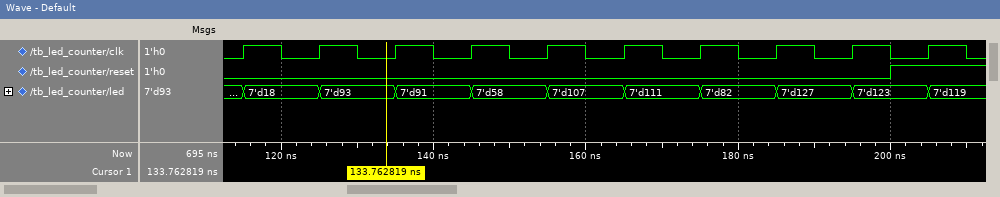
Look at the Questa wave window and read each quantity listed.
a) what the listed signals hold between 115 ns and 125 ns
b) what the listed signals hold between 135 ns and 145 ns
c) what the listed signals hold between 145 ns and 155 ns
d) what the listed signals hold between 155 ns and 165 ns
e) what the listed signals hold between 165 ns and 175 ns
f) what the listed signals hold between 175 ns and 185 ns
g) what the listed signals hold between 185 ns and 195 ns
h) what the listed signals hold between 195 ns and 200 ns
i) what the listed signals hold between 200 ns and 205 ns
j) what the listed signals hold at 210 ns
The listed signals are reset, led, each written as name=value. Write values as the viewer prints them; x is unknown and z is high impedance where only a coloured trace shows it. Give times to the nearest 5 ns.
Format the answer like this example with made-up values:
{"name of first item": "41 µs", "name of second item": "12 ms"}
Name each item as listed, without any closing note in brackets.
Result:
{"what the listed signals hold between 115 ns and 125 ns": "reset=0, led=7'd18", "what the listed signals hold between 135 ns and 145 ns": "reset=0, led=7'd91", "what the listed signals hold between 145 ns and 155 ns": "reset=0, led=7'd58", "what the listed signals hold between 155 ns and 165 ns": "reset=0, led=7'd107", "what the listed signals hold between 165 ns and 175 ns": "reset=0, led=7'd111", "what the listed signals hold between 175 ns and 185 ns": "reset=0, led=7'd82", "what the listed signals hold between 185 ns and 195 ns": "reset=0, led=7'd127", "what the listed signals hold between 195 ns and 200 ns": "reset=0, led=7'd123", "what the listed signals hold between 200 ns and 205 ns": "reset=1, led=7'd123", "what the listed signals hold at 210 ns": "reset=1, led=7'd119"}
